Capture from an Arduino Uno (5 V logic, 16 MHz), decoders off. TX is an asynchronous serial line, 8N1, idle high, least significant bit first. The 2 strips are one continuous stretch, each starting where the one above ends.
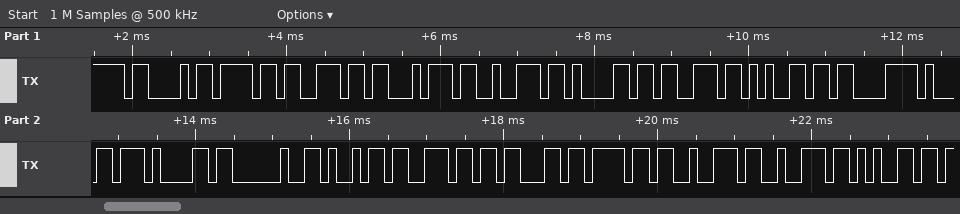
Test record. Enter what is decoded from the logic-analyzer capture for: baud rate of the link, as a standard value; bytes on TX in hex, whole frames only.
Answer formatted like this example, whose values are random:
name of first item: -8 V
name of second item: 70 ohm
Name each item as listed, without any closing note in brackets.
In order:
baud rate of the link, as a standard value: 9600 baud
bytes on TX in hex, whole frames only: 0x43 0x6F 0x6E 0x74 0x72 0x61 0x73 0x65 0xC3 0xB1 0x61 0x20 0x69 0x6E 0x63 0x6F 0x72 0x72 0x65
